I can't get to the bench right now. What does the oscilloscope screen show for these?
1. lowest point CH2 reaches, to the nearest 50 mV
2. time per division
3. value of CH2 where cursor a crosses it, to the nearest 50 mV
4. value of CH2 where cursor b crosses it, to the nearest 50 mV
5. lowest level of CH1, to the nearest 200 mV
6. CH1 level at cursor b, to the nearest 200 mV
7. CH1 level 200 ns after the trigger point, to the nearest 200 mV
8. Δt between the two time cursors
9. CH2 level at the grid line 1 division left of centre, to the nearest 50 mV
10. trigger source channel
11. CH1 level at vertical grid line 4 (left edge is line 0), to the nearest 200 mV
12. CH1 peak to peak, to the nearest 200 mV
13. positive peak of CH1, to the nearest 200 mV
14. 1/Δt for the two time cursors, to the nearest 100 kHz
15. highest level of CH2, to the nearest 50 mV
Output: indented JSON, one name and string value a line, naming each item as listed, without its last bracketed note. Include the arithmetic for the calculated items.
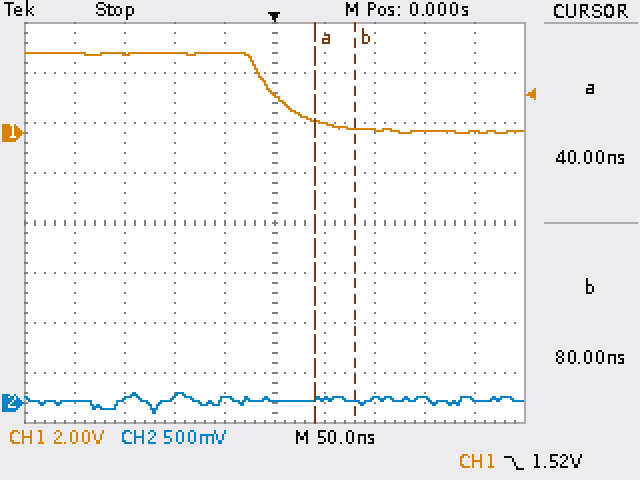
{
  "lowest point CH2 reaches, to the nearest 50 mV": "-100 mV",
  "time per division": "50 ns",
  "value of CH2 where cursor a crosses it, to the nearest 50 mV": "50 mV",
  "value of CH2 where cursor b crosses it, to the nearest 50 mV": "0 mV",
  "lowest level of CH1, to the nearest 200 mV": "0.0 V",
  "CH1 level at cursor b, to the nearest 200 mV": "200 mV",
  "CH1 level 200 ns after the trigger point, to the nearest 200 mV": "0.0 V",
  "Δt between the two time cursors": "80 ns − (40 ns) = 40 ns",
  "CH2 level at the grid line 1 division left of centre, to the nearest 50 mV": "50 mV",
  "trigger source channel": "CH1",
  "CH1 level at vertical grid line 4 (left edge is line 0), to the nearest 200 mV": "3.2 V",
  "CH1 peak to peak, to the nearest 200 mV": "3.2 V − (0.0 V) = 3.2 V",
  "positive peak of CH1, to the nearest 200 mV": "3.2 V",
  "1/Δt for the two time cursors, to the nearest 100 kHz": "1 / 40 ns ≈ 25.0 MHz",
  "highest level of CH2, to the nearest 50 mV": "100 mV"
}
